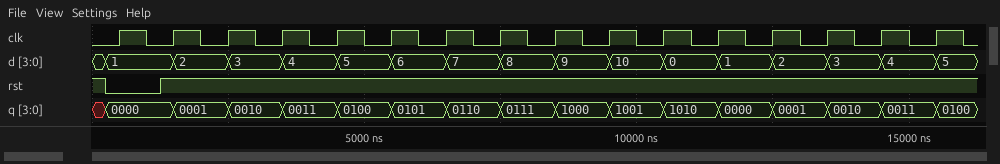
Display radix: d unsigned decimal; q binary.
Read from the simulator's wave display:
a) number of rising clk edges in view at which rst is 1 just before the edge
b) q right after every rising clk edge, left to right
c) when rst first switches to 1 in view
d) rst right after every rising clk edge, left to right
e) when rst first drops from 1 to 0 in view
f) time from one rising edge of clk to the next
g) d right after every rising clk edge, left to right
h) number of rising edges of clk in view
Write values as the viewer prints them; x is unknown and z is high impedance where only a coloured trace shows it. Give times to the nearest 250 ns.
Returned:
15
0000, 0001, 0010, 0011, 0100, 0101, 0110, 0111, 1000, 1001, 1010, 0000, 0001, 0010, 0011, 0100
1250 ns
0 1 1 1 1 1 1 1 1 1 1 1 1 1 1 1
250 ns
1000 ns
1, 2, 3, 4, 5, 6, 7, 8, 9, 10, 0, 1, 2, 3, 4, 5
16
